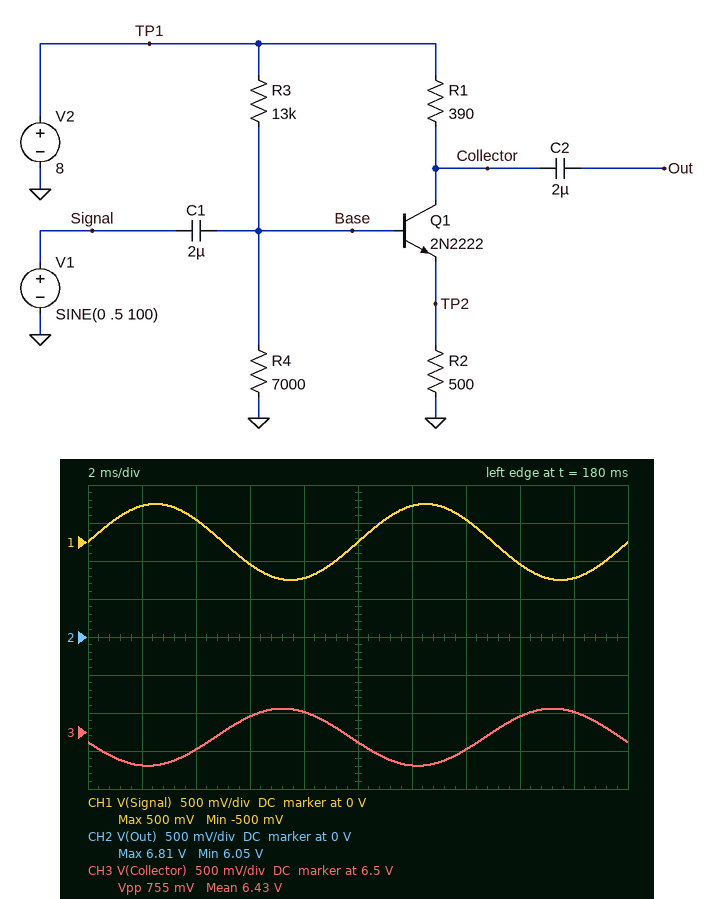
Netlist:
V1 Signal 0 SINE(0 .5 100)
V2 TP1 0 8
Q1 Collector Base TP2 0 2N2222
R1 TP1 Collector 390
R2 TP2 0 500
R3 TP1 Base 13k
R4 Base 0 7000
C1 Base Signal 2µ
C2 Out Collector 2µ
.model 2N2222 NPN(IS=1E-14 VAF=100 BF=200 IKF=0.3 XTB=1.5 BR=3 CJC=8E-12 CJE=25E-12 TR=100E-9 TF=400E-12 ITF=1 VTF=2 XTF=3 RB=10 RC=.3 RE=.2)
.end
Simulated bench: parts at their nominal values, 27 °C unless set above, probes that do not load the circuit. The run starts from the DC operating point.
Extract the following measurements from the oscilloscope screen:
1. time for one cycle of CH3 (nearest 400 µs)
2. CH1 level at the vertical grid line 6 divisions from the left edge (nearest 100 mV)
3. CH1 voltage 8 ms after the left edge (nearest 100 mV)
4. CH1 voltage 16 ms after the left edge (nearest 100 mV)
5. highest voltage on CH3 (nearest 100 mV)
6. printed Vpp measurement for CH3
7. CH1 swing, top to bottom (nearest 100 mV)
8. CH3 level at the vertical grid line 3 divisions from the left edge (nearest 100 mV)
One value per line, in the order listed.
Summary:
10.0 ms
500 mV
-500 mV
-300 mV
6.8 V
755 mV
1.0 V
6.7 V
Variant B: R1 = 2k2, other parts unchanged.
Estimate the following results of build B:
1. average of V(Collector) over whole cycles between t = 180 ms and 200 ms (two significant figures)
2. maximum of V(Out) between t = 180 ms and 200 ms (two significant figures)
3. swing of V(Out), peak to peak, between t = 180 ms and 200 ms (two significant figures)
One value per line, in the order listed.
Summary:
2.4 V
3.8 V
2.2 V
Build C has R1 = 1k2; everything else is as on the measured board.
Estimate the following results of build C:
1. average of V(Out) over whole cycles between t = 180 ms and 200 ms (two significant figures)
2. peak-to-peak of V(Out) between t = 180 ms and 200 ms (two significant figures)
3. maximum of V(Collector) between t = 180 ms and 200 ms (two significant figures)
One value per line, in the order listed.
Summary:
3.4 V
2.1 V
4.5 V
